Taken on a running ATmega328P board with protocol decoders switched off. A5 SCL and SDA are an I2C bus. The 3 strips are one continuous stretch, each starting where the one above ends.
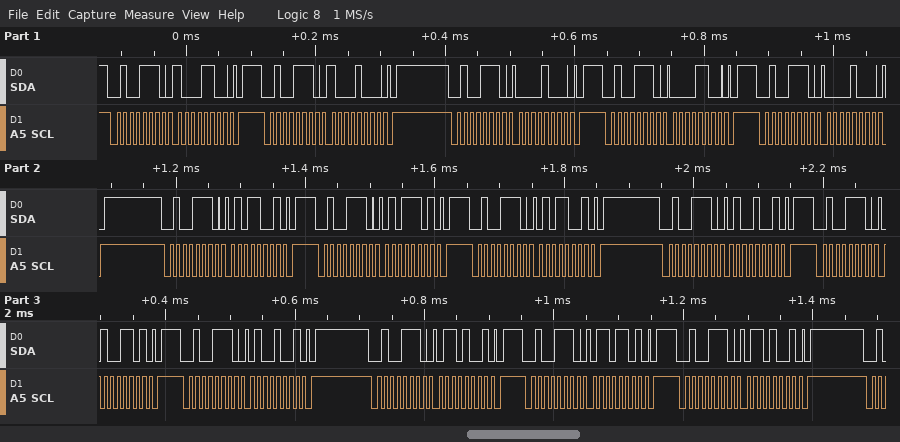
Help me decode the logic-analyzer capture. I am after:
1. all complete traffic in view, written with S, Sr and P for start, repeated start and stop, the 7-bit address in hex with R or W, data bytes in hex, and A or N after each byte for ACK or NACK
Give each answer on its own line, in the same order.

S 27W A 8C A P S 27W A 88 A P S 27W A 08 A P S 27W A 0C A P S 27W A 08 A P S 27W A 59 A P S 27W A 5D A P S 27W A 59 A P S 27W A 49 A P S 27W A 4D A P S 27W A 49 A P S 27W A 69 A P S 27W A 6D A P S 27W A 69 A P
